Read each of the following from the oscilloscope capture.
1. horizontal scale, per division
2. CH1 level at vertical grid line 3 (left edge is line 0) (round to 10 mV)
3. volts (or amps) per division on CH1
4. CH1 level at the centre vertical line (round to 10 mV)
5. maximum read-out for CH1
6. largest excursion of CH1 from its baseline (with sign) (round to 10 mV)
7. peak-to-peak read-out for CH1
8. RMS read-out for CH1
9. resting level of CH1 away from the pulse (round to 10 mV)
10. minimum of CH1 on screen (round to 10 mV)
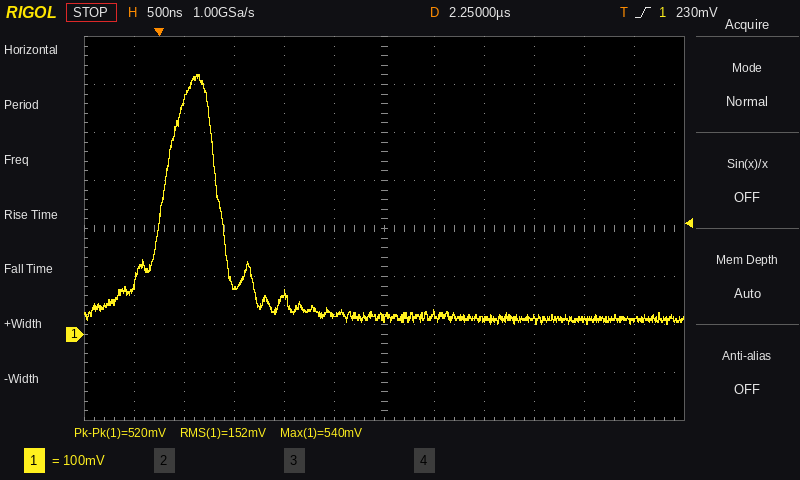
500 ns
100 mV
100 mV
30 mV
540 mV
+510 mV
520 mV
152 mV
30 mV
20 mV
